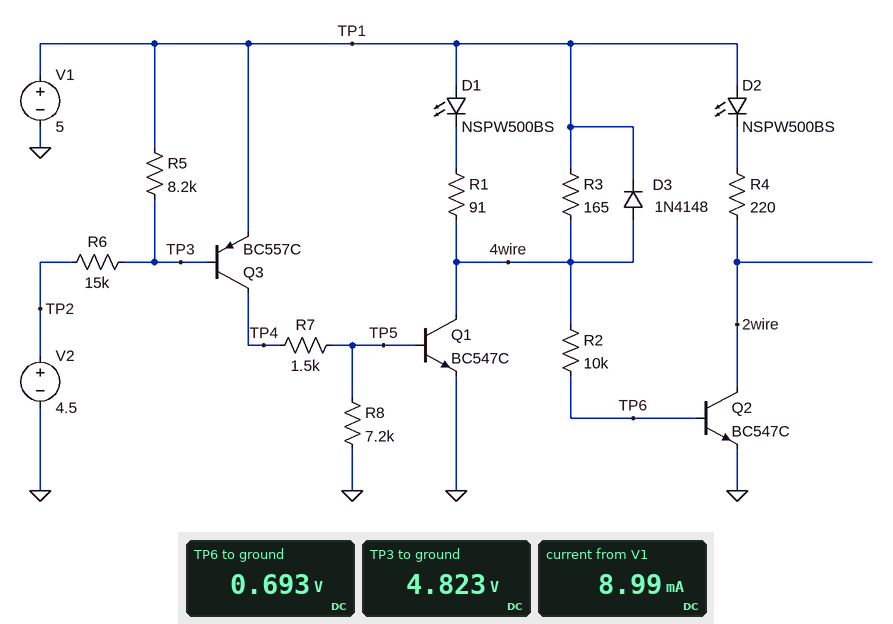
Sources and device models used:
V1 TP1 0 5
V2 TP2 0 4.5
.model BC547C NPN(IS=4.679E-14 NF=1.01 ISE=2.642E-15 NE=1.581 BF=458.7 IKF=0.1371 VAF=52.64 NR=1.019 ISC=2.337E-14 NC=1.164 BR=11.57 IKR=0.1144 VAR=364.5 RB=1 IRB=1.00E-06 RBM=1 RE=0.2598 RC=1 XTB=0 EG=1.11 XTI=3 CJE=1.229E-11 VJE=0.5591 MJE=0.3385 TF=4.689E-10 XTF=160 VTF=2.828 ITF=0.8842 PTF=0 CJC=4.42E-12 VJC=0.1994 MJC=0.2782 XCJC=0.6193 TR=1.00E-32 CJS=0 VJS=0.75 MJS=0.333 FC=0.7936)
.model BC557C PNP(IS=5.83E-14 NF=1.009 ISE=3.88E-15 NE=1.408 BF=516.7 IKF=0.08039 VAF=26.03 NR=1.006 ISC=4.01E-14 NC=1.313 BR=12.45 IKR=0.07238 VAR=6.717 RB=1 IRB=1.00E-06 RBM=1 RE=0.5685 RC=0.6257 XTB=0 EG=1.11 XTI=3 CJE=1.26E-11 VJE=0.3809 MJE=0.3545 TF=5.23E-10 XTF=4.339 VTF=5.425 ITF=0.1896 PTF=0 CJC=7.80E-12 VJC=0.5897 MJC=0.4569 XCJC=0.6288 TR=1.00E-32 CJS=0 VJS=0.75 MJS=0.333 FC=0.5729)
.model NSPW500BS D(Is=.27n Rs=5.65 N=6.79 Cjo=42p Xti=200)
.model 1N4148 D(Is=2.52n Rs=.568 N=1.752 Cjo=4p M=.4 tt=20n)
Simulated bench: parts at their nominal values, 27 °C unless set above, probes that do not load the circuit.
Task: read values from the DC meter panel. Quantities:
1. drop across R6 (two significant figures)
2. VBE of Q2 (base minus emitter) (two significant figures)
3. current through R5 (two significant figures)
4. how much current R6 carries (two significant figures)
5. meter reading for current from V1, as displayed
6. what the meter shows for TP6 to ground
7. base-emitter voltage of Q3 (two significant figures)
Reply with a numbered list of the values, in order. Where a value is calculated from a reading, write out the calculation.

1. 4.823 V - 4.5 V = 320 mV
2. 693 mV = 690 mV
3. (5 V - 4.823 V) / 8.2 kΩ = 22 µA
4. (4.823 V - 4.5 V) / 15 kΩ = 22 µA
5. 8.99 mA
6. 0.693 V
7. 4.823 V - 5 V = -180 mV
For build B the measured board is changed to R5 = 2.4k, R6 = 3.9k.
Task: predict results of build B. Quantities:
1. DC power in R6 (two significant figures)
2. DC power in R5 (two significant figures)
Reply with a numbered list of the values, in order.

1. 25 µW
2. 15 µW
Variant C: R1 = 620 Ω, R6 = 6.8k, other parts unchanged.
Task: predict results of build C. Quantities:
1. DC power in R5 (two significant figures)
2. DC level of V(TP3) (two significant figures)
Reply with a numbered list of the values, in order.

1. 9.1 µW
2. 4.7 V
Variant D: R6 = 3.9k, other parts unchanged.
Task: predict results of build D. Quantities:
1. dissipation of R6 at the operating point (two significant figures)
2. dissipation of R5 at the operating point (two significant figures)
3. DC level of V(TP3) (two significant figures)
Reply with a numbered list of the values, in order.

1. 6.7 µW
2. 14 µW
3. 4.7 V
